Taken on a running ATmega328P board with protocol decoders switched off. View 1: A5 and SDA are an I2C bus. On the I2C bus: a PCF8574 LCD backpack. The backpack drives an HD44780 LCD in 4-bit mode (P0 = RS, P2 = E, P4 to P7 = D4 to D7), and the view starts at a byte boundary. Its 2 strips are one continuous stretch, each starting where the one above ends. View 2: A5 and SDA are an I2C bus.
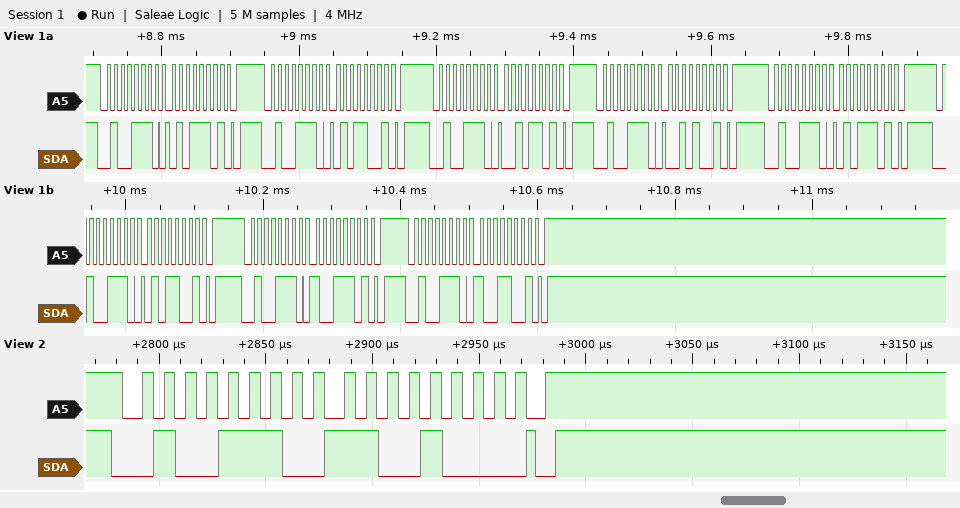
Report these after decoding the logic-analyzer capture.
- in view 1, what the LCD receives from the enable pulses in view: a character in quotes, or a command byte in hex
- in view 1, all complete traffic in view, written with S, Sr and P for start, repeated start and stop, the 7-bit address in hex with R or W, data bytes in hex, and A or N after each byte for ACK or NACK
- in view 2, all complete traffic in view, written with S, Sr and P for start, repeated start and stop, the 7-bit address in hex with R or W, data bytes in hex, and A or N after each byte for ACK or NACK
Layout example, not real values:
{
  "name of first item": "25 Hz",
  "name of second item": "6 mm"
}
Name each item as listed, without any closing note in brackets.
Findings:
{
  "in view 1, what the LCD receives from the enable pulses in view: a character in quotes, or a command byte in hex": "'R' 'Y'",
  "in view 1, all complete traffic in view, written with S, Sr and P for start, repeated start and stop, the 7-bit address in hex with R or W, data bytes in hex, and A or N after each byte for ACK or NACK": "S 27W A 5D A P S 27W A 59 A P S 27W A 2D A P S 27W A 29 A P S 27W A 5D A P S 27W A 59 A P S 27W A 9D A P S 27W A 99 A P",
  "in view 2, all complete traffic in view, written with S, Sr and P for start, repeated start and stop, the 7-bit address in hex with R or W, data bytes in hex, and A or N after each byte for ACK or NACK": "S 27W A C8 A P"
}
